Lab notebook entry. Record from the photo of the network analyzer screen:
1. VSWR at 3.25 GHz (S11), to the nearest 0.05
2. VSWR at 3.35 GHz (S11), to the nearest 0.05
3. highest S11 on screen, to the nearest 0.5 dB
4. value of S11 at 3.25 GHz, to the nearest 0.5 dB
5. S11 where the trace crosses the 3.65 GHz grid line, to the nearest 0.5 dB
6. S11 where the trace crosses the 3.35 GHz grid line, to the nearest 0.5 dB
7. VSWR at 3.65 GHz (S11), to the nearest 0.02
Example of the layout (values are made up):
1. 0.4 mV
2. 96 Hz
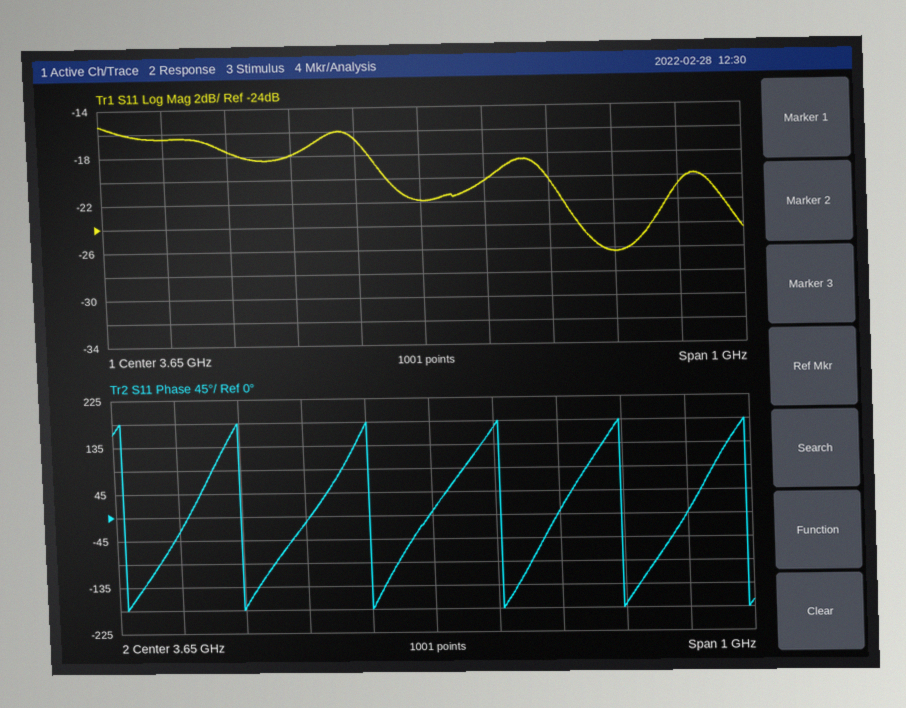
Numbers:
1. 1.35
2. 1.30
3. -15.5 dB
4. -16.5 dB
5. -22.0 dB
6. -17.5 dB
7. 1.18
